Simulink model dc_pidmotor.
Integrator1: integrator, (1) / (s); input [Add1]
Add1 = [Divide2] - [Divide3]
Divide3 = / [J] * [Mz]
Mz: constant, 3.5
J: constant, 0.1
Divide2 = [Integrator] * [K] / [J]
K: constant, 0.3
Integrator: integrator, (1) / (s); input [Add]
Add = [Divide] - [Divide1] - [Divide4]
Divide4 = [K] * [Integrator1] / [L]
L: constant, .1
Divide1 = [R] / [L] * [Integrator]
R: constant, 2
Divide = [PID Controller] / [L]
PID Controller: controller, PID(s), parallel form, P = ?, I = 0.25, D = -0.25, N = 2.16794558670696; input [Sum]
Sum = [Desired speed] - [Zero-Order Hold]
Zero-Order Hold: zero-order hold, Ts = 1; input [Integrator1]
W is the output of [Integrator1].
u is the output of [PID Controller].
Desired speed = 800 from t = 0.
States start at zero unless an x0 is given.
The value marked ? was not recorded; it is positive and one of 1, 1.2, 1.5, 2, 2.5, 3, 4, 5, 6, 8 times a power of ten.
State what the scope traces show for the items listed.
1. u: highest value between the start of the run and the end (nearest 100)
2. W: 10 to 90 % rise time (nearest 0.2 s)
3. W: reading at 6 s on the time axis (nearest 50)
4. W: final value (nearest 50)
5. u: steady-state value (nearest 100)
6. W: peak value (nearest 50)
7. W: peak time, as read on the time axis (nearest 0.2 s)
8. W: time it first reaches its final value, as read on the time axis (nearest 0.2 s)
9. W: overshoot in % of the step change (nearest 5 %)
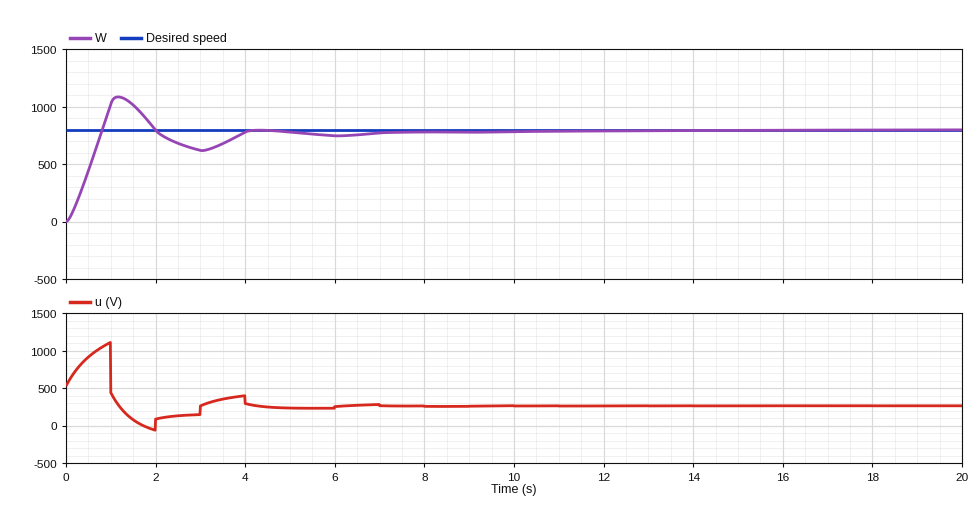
1100
0.6 s
750
800
300
1100
1.2 s
0.8 s
35 %
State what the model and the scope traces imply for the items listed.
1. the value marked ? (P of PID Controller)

1.2
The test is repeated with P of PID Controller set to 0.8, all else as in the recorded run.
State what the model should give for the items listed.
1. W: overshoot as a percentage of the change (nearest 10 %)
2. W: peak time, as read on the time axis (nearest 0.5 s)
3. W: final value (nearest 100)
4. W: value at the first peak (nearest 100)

20 %
2.0 s
800
1000
